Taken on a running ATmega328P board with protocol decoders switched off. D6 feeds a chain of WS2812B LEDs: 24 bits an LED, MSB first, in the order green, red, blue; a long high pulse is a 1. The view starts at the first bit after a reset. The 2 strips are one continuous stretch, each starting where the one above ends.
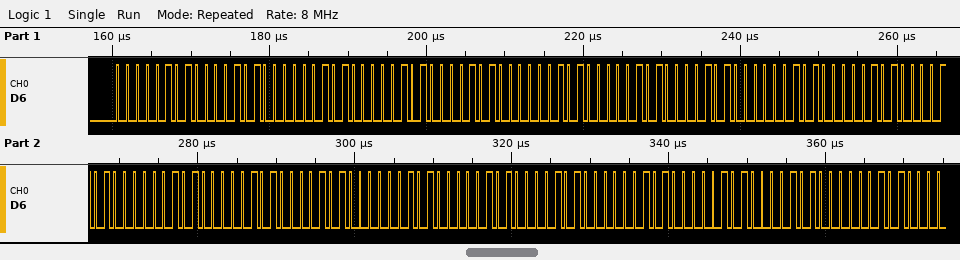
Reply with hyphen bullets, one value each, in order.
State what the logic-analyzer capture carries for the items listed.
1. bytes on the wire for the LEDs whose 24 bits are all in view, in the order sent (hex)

- 05 0A 05 05 0A 05 05 0A 05 05 0A 05 05 0A 05 05 0A 05 05 0A 05
